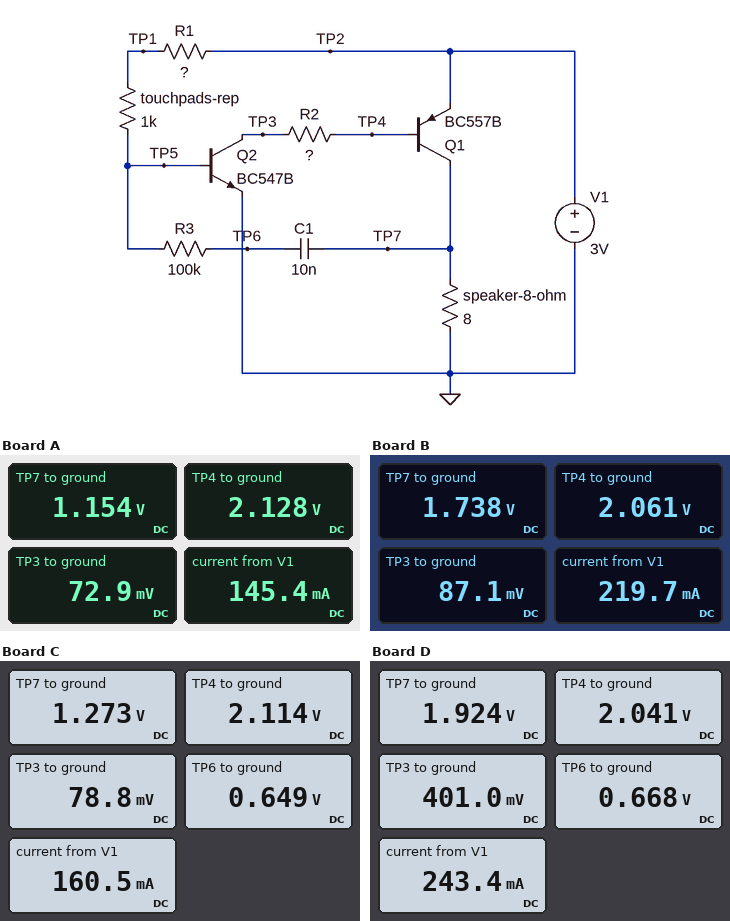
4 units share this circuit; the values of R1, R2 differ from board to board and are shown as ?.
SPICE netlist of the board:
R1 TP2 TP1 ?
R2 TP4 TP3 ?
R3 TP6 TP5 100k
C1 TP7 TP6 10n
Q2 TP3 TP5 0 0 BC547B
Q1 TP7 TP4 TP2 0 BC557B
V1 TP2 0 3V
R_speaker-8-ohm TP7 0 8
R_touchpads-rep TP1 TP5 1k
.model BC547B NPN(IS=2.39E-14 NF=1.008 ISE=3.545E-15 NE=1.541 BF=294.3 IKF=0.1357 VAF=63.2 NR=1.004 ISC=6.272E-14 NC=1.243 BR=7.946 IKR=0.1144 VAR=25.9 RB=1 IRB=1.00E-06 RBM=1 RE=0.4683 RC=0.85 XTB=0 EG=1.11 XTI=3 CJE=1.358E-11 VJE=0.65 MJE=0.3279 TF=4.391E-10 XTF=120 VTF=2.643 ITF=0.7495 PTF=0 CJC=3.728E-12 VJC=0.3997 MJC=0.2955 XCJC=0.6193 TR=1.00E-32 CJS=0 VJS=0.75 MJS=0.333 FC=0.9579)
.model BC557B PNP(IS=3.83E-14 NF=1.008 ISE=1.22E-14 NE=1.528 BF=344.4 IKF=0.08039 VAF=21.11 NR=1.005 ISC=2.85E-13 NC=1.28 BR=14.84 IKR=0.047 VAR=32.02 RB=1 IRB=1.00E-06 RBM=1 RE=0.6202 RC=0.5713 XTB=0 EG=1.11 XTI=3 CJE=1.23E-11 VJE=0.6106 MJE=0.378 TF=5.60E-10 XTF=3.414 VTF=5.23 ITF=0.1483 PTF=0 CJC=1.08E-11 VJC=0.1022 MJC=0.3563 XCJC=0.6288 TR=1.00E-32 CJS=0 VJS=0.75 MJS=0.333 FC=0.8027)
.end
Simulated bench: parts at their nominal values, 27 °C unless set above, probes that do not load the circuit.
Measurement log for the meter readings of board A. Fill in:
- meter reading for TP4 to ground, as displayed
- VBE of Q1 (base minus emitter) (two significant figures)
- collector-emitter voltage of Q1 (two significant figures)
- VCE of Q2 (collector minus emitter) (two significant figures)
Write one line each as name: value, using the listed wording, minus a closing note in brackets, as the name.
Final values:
meter reading for TP4 to ground, as displayed: 2.128 V
VBE of Q1 (base minus emitter): -870 mV
collector-emitter voltage of Q1: -1.8 V
VCE of Q2 (collector minus emitter): 73 mV
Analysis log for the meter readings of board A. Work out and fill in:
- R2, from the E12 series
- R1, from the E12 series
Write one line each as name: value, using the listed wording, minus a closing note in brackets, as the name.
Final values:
R2, from the E12 series: 1.8 kΩ
R1, from the E12 series: 120 kΩ
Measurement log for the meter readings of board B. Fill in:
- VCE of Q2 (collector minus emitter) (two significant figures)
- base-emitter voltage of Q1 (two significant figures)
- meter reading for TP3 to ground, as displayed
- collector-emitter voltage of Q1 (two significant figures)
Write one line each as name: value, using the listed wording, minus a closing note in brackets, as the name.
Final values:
VCE of Q2 (collector minus emitter): 87 mV
base-emitter voltage of Q1: -940 mV
meter reading for TP3 to ground, as displayed: 87.1 mV
collector-emitter voltage of Q1: -1.3 V
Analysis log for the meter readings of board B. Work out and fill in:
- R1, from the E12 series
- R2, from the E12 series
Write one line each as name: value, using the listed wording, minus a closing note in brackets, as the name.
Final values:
R1, from the E12 series: 82 kΩ
R2, from the E12 series: 820 Ω
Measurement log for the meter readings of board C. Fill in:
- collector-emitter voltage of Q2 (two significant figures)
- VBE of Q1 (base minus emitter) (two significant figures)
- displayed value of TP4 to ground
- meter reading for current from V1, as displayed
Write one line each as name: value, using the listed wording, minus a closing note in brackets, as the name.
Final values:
collector-emitter voltage of Q2: 79 mV
VBE of Q1 (base minus emitter): -890 mV
displayed value of TP4 to ground: 2.114 V
meter reading for current from V1, as displayed: 160.5 mA
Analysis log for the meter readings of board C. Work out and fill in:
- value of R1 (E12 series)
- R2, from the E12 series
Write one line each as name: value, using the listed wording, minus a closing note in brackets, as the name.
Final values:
value of R1: 120 kΩ
R2, from the E12 series: 1.5 kΩ
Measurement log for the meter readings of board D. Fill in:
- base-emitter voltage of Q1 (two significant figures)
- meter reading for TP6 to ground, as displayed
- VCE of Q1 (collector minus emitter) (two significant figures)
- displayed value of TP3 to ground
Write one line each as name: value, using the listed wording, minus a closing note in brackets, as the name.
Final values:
base-emitter voltage of Q1: -960 mV
meter reading for TP6 to ground, as displayed: 0.668 V
VCE of Q1 (collector minus emitter): -1.1 V
displayed value of TP3 to ground: 401.0 mV
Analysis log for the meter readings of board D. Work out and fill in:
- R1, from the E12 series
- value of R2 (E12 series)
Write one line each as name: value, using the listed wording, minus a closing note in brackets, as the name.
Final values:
R1, from the E12 series: 220 kΩ
value of R2: 560 Ω
